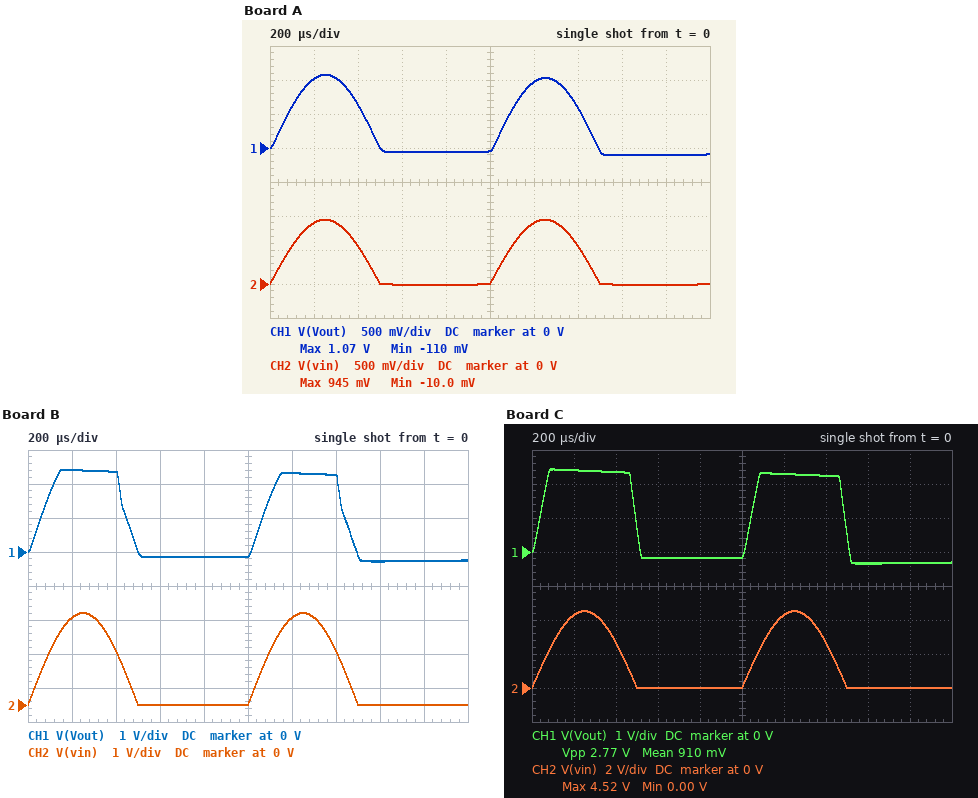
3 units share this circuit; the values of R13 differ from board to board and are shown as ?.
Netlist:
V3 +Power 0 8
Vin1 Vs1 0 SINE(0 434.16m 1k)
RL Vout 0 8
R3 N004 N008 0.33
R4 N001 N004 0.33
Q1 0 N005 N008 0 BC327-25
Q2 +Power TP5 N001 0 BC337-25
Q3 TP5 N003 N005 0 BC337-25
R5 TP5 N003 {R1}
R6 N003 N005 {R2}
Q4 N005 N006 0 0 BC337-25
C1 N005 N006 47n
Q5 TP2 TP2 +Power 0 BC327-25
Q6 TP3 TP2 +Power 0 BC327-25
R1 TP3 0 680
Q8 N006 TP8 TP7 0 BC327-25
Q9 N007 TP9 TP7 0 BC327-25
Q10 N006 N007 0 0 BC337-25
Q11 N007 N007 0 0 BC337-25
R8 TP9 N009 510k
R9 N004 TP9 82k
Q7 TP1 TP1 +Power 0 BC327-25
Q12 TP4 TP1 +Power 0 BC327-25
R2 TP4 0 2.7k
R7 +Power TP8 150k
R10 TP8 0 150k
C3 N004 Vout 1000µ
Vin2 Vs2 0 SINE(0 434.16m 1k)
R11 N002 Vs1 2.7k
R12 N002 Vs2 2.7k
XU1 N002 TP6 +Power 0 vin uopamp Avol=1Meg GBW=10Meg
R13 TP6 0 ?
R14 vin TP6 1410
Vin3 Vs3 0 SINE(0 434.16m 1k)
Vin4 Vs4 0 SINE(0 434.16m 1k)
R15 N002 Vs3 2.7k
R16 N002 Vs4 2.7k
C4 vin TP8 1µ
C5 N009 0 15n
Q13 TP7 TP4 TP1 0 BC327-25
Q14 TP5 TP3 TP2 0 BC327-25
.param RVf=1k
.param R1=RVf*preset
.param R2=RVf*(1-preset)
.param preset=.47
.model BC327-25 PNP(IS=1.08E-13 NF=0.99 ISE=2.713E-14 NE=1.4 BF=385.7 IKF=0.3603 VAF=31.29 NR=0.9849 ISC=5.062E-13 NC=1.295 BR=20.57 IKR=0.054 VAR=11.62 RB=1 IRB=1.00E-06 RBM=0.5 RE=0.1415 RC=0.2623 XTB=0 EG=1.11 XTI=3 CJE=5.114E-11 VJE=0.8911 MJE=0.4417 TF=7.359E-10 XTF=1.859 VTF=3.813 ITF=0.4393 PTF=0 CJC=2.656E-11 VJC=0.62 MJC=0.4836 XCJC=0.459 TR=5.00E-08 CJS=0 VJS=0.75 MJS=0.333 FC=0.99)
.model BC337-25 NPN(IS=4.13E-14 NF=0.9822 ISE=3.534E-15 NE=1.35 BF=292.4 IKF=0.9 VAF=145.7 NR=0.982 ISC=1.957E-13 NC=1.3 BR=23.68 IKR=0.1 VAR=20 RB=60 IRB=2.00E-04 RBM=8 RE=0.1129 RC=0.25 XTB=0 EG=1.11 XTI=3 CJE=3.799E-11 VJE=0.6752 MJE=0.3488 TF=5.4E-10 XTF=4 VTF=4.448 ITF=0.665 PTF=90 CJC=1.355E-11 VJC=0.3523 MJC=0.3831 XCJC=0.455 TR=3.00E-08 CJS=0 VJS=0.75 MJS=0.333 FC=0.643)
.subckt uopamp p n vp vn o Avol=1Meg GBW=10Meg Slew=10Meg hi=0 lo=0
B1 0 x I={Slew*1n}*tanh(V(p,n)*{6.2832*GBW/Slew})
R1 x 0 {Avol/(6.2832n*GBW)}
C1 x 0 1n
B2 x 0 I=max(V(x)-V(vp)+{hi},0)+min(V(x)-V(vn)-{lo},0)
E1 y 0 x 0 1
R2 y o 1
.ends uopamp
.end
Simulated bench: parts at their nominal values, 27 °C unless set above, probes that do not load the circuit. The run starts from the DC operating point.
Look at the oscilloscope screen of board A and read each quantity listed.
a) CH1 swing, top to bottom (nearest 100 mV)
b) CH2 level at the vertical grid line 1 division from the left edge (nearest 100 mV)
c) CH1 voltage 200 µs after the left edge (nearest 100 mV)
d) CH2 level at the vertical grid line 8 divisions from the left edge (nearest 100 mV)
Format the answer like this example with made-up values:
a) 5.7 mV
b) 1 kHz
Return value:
a) 1.2 V
b) 900 mV
c) 1.0 V
d) 0 V
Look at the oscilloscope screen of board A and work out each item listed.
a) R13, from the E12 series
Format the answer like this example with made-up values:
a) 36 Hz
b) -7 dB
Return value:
a) 1.2 kΩ
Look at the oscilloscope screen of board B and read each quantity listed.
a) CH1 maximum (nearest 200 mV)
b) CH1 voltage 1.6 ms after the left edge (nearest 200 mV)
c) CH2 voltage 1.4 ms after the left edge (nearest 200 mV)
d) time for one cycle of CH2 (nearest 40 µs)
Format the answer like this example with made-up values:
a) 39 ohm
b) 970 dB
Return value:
a) 2.4 V
b) -200 mV
c) 1.6 V
d) 1.00 ms
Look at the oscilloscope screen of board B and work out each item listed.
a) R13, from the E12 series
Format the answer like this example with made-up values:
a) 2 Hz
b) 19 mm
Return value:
a) 270 Ω
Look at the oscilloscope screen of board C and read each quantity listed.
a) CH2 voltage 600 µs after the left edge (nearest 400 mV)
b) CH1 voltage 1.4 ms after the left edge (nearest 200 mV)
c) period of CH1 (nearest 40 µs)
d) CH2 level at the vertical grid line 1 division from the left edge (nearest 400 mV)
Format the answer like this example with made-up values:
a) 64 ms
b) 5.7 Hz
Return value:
a) 0 V
b) 2.2 V
c) 1.00 ms
d) 4.4 V
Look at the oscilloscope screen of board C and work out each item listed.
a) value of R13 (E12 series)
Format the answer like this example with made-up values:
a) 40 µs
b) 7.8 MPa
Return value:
a) 150 Ω
